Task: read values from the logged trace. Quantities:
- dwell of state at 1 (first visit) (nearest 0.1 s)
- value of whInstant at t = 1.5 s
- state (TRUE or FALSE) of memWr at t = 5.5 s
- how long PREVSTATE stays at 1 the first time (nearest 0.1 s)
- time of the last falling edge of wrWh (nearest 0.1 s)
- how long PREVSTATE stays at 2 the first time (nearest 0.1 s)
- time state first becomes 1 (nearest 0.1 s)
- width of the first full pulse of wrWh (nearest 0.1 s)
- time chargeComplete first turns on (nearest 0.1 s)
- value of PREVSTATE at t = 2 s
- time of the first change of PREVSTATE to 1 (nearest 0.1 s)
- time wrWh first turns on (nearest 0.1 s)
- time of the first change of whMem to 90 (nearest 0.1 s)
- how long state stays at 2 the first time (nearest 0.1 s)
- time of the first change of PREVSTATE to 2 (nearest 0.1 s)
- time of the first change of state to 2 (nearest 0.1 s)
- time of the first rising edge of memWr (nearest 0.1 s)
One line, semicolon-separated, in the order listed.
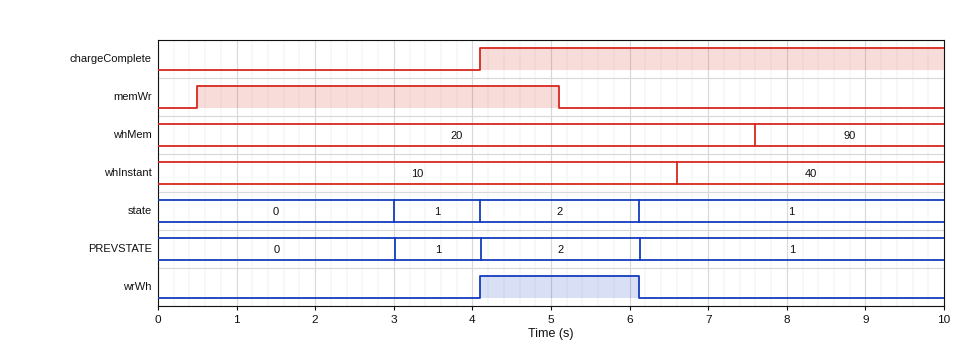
1.1 s; 10; FALSE; 1.1 s; 6.1 s; 2.0 s; 3.0 s; 2.0 s; 4.1 s; 0; 3.0 s; 4.1 s; 7.6 s; 2.0 s; 4.1 s; 4.1 s; 0.5 s
